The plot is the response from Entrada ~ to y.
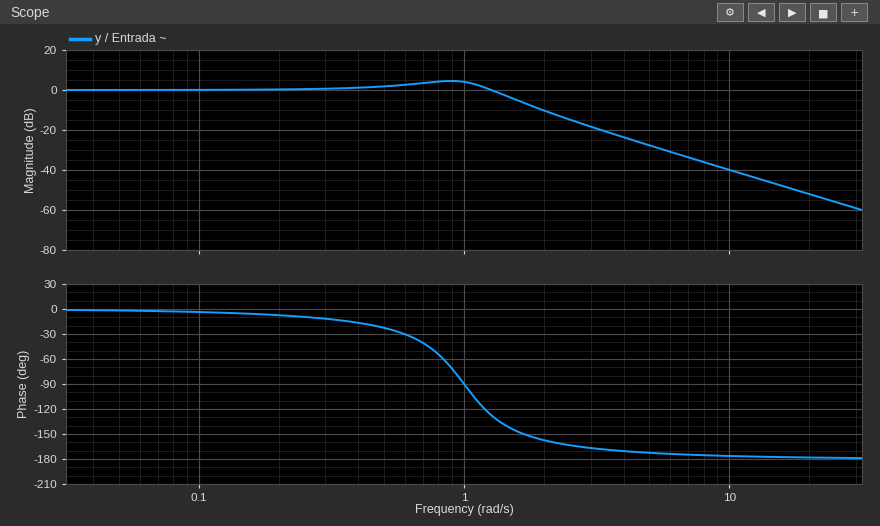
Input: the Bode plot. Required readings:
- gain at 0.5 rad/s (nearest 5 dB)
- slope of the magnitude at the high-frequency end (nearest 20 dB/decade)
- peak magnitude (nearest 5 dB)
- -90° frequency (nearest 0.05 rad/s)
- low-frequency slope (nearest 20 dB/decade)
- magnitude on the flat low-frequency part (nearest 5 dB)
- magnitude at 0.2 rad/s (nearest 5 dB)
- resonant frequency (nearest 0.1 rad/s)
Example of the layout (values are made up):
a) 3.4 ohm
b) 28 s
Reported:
a) 0 dB
b) -40 dB/decade
c) 5 dB
d) 1.00 rad/s
e) 0 dB/decade
f) 0 dB
g) 0 dB
h) 0.9 rad/s
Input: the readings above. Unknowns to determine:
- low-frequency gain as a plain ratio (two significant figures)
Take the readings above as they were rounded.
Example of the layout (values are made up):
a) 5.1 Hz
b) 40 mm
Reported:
a) 1.0
